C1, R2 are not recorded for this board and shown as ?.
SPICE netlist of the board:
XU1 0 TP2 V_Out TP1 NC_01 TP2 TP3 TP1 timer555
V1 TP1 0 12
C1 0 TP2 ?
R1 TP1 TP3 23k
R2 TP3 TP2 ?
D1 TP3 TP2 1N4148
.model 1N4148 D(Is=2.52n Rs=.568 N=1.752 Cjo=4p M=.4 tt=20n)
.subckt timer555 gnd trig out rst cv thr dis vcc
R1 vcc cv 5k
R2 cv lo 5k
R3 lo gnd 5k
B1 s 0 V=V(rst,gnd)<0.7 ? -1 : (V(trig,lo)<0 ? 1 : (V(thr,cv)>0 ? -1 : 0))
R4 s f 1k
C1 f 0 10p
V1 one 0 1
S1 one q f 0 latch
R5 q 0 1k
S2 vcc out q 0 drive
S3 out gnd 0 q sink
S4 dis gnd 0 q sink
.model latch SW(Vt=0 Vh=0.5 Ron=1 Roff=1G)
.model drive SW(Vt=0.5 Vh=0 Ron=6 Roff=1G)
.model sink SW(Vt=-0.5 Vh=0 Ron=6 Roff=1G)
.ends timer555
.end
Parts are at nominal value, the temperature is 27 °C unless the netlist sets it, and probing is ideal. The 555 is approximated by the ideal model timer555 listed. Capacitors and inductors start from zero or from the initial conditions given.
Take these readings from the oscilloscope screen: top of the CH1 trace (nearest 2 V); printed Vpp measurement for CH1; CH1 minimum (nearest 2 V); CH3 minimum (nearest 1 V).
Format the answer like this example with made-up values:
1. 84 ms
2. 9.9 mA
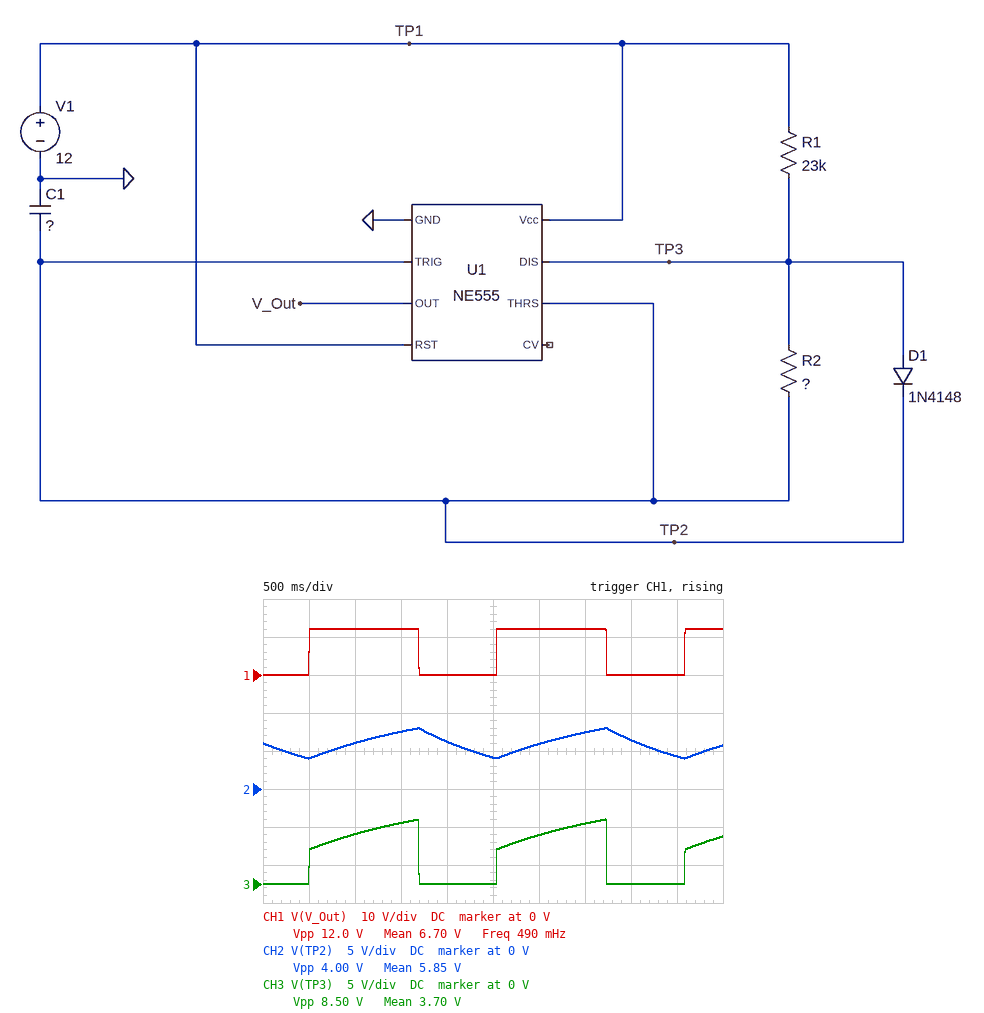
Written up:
1. 12 V
2. 12.0 V
3. 0 V
4. 0 V
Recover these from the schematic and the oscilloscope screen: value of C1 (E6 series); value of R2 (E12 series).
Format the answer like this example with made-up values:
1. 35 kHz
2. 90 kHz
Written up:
1. 68 µF
2. 18 kΩ
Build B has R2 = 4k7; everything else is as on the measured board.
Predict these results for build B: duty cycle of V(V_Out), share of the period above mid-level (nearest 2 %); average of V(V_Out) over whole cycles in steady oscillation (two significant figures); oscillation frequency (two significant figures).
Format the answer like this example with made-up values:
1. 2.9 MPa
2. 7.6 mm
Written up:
1. 84 %
2. 10 V
3. 710 mHz
